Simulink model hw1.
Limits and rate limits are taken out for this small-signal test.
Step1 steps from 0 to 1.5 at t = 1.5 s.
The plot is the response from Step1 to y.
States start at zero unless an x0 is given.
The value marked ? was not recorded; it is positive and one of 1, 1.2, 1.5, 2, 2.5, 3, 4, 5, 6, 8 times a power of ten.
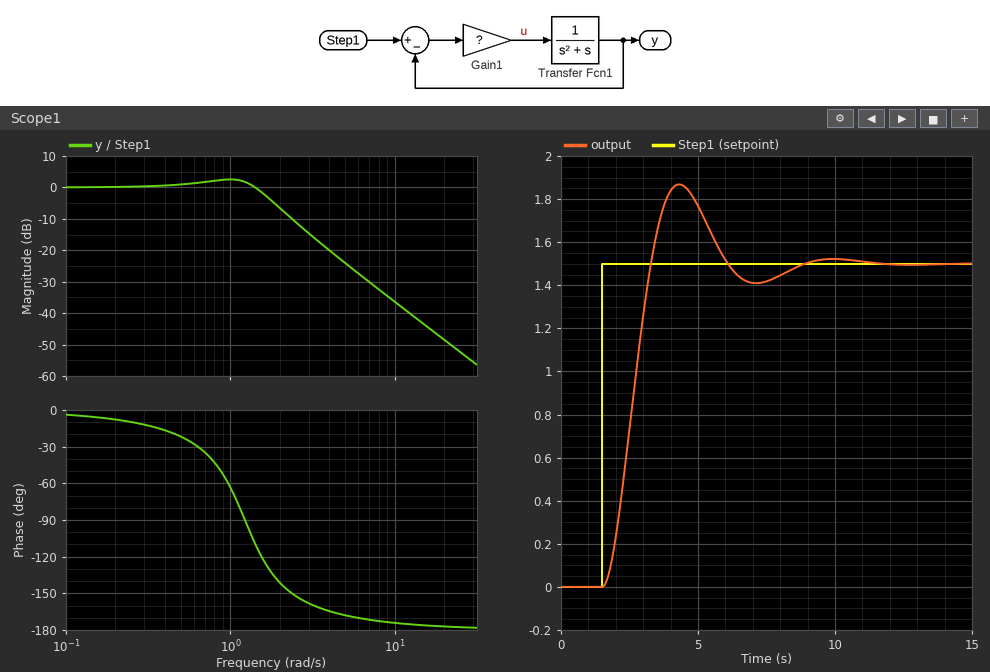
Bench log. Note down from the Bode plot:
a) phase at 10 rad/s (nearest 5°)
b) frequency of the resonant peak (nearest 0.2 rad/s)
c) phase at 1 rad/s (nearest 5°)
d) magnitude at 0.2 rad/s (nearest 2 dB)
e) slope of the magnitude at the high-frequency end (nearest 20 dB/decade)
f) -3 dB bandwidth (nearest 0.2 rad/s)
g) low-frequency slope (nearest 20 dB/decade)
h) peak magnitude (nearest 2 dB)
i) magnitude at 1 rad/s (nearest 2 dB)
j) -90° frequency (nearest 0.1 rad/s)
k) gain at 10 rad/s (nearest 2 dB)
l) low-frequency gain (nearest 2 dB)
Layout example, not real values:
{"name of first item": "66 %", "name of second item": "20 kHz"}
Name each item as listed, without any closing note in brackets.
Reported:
{"phase at 10 rad/s": "-175°", "frequency of the resonant peak": "1.0 rad/s", "phase at 1 rad/s": "-65°", "magnitude at 0.2 rad/s": "0 dB", "slope of the magnitude at the high-frequency end": "-40 dB/decade", "-3 dB bandwidth": "1.6 rad/s", "low-frequency slope": "0 dB/decade", "peak magnitude": "2 dB", "magnitude at 1 rad/s": "2 dB", "-90° frequency": "1.2 rad/s", "gain at 10 rad/s": "-36 dB", "low-frequency gain": "0 dB"}
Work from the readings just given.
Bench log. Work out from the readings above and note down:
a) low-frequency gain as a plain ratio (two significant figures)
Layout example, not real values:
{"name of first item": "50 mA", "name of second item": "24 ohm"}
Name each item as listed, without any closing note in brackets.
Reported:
{"low-frequency gain as a plain ratio": "1.0"}
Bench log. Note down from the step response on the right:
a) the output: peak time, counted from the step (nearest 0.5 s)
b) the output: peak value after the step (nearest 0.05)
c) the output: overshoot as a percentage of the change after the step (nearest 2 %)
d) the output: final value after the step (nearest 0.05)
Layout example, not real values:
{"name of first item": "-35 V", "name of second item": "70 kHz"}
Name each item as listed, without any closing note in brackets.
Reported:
{"the output: peak time, counted from the step": "3.0 s", "the output: peak value after the step": "1.85", "the output: overshoot as a percentage of the change after the step": "24 %", "the output: final value after the step": "1.50"}
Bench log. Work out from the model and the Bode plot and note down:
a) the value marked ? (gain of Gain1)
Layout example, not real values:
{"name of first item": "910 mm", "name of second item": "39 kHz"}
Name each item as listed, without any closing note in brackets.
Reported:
{"the value marked ?": "1.5"}
